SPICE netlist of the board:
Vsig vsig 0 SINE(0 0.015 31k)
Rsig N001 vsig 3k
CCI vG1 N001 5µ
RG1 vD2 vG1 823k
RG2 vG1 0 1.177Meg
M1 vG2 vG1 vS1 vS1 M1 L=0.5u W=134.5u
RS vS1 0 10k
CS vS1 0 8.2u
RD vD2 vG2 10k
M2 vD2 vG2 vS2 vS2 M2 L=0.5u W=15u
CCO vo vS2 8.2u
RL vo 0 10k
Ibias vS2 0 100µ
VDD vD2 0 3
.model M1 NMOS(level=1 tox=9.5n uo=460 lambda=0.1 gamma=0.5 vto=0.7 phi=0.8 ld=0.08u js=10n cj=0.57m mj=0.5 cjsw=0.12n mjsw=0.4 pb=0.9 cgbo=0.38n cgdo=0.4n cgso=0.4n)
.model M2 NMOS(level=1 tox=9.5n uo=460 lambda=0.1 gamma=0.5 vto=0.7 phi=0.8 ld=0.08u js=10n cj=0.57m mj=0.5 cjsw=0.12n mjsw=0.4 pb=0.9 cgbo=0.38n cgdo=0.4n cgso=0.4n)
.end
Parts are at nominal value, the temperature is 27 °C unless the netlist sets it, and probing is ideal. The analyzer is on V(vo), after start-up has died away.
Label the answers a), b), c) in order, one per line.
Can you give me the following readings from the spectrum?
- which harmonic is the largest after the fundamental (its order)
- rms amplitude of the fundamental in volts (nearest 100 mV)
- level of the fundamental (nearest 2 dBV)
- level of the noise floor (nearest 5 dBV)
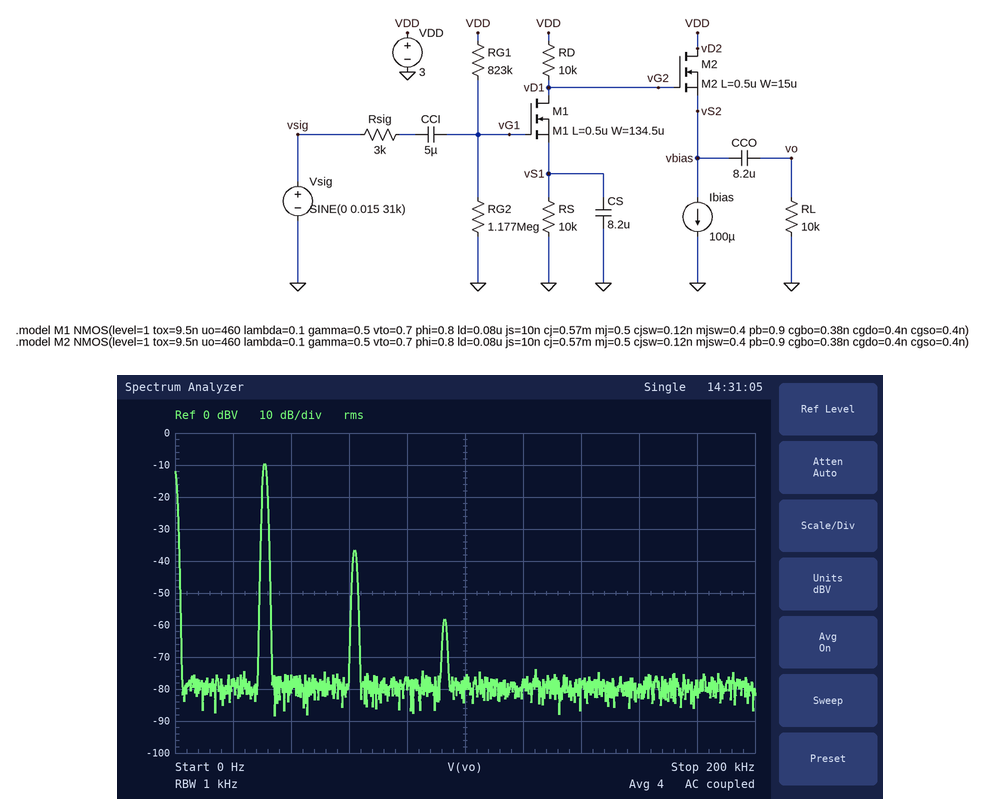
a) 2
b) 300 mV
c) -10 dBV
d) -80 dBV
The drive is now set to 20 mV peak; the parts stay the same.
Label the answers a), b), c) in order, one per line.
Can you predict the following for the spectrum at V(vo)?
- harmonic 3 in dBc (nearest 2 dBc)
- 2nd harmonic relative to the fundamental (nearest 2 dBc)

a) -44 dBc
b) -24 dBc
